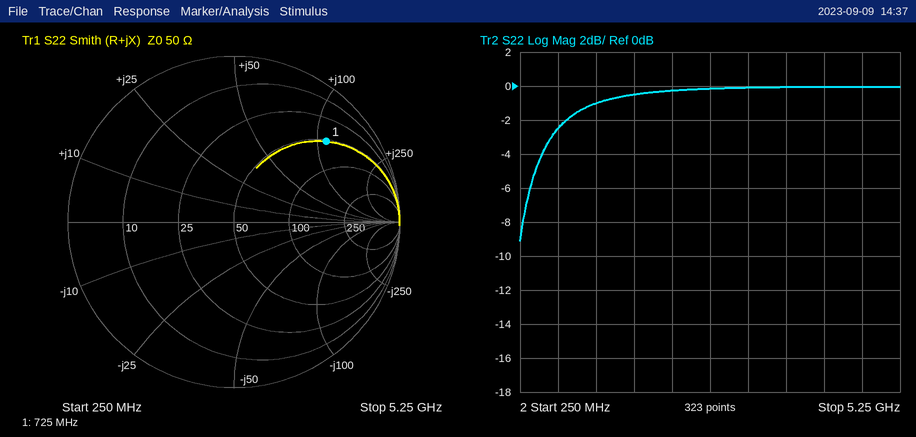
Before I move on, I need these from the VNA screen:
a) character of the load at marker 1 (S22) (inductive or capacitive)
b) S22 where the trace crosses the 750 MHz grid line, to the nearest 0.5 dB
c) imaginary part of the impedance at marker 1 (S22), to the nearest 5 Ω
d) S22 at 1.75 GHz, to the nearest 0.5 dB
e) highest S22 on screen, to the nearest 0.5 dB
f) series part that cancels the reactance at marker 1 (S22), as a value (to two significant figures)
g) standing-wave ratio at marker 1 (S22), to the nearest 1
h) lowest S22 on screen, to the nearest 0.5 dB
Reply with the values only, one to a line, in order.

inductive
-2.5 dB
+110 Ω
-0.5 dB
0.0 dB
2.0 pF
7
-9.0 dB
